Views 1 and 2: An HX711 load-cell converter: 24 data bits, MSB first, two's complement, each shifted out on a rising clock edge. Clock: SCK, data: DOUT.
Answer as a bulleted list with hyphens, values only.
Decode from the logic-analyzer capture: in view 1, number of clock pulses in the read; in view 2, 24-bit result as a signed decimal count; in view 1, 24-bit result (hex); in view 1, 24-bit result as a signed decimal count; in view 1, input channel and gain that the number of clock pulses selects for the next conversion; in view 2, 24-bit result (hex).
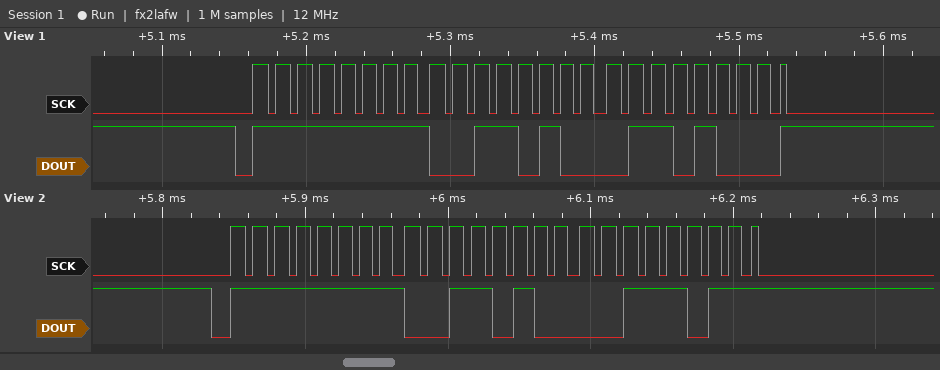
- 25
- -52165
- 0xFF3468
- -52120
- channel A, gain 128
- 0xFF343B
